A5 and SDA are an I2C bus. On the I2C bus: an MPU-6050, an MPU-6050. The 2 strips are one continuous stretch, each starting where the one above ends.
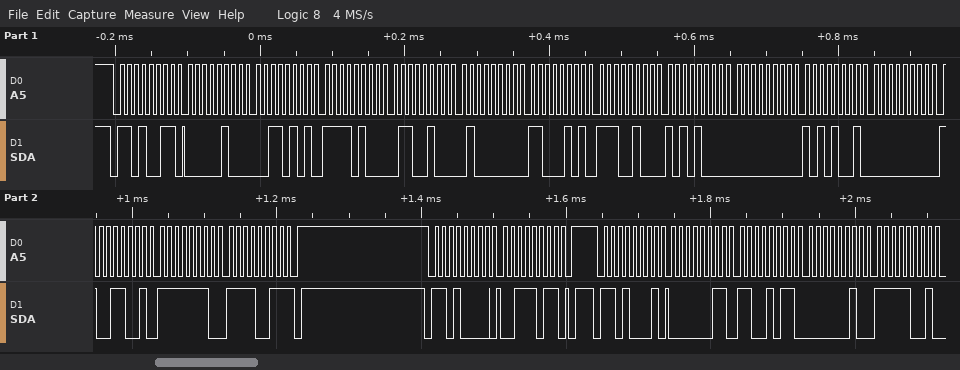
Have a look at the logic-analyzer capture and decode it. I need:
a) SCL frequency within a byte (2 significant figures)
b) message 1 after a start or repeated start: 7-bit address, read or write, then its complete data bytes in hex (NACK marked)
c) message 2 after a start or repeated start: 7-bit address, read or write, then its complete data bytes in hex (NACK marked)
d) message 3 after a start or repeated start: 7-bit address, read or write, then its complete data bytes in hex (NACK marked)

100 kHz
0x69 read: 04 35 F4 64 40 C5 E4 A8 00 A9 00 99 FE F3 NACK
0x68 write: 3B
0x68 read: 03 CB 02 F9
